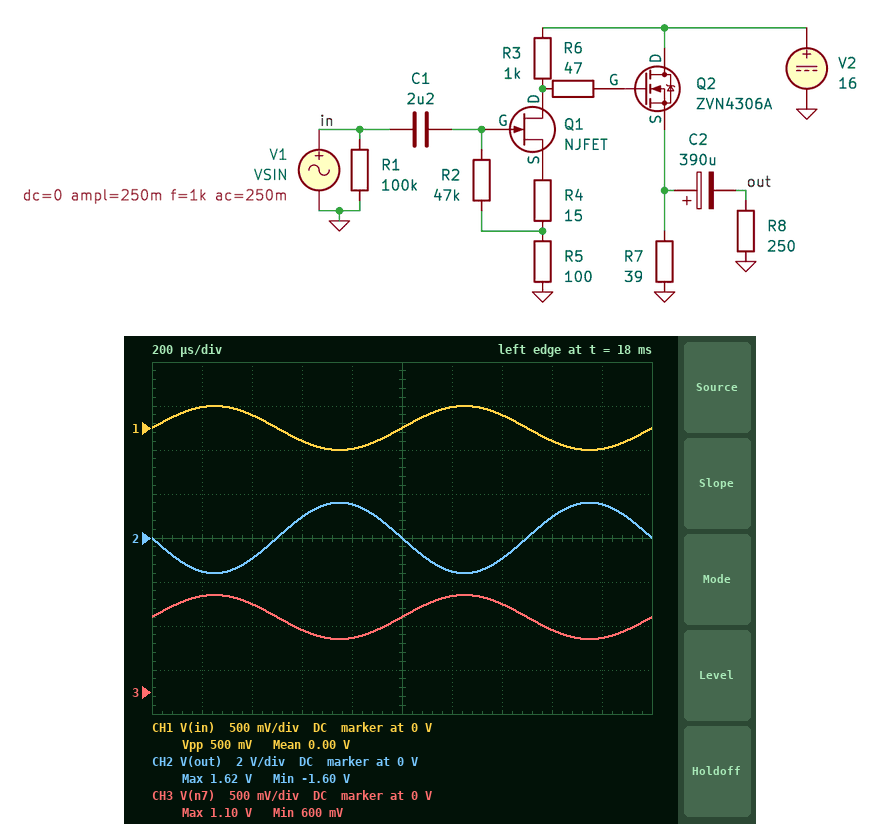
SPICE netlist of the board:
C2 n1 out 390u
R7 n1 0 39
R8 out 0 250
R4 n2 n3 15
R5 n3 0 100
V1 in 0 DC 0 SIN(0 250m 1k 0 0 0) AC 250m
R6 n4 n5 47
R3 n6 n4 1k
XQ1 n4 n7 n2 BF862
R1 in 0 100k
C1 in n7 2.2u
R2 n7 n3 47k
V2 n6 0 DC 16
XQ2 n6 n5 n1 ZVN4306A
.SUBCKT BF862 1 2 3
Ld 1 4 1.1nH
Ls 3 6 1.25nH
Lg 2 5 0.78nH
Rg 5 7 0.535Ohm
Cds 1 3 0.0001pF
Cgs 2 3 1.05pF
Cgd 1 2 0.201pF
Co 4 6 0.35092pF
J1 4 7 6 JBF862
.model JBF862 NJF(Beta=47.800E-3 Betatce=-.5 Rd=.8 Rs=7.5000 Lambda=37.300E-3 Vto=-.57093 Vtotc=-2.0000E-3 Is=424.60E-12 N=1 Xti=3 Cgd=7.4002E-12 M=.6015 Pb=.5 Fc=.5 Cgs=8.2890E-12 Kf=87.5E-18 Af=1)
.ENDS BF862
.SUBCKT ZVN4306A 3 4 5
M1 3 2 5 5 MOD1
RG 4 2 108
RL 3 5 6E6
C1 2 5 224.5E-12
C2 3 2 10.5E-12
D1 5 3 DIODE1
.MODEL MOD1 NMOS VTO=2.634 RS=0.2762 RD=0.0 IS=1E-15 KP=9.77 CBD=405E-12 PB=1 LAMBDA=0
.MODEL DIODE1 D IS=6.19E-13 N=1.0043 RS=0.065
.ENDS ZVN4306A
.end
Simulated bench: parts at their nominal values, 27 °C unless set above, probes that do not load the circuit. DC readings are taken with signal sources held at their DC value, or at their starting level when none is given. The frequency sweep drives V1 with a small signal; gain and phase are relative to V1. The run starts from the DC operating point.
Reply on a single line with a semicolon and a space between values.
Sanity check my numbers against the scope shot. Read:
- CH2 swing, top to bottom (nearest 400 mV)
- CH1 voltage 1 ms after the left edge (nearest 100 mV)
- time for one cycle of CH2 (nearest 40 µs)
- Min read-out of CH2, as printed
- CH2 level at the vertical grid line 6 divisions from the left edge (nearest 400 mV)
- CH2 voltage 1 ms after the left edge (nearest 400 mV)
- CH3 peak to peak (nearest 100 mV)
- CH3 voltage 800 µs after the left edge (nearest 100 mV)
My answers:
3.2 V; 0 V; 1.00 ms; -1.60 V; -1.6 V; 0 V; 500 mV; 600 mV
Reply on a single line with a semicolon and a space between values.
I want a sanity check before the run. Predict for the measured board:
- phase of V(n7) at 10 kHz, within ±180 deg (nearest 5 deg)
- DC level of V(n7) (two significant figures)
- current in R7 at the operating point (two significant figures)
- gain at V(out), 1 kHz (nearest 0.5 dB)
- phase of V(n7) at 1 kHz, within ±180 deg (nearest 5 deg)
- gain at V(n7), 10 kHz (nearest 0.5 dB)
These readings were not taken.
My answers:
0 deg; 850 mV; 120 mA; 16.0 dB; 0 deg; 0 dB
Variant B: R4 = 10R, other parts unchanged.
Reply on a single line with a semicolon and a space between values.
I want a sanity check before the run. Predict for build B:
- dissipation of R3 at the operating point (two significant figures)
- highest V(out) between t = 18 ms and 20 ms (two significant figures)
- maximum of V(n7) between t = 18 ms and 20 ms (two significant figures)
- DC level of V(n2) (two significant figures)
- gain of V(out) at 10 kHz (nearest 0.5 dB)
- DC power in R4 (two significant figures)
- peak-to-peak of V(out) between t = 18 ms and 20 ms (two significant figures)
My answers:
89 mW; 1.7 V; 1.2 V; 1.0 V; 16.5 dB; 890 µW; 3.3 V
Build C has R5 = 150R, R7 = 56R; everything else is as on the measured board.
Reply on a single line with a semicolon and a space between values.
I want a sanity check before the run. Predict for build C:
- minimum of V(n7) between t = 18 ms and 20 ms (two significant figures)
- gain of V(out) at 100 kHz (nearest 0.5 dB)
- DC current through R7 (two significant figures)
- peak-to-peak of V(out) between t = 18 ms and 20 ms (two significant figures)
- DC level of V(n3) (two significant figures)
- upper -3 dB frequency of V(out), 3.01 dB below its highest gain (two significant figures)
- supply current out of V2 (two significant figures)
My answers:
1.0 V; 13.5 dB; 85 mA; 2.4 V; 1.3 V; 8.8 MHz; 93 mA
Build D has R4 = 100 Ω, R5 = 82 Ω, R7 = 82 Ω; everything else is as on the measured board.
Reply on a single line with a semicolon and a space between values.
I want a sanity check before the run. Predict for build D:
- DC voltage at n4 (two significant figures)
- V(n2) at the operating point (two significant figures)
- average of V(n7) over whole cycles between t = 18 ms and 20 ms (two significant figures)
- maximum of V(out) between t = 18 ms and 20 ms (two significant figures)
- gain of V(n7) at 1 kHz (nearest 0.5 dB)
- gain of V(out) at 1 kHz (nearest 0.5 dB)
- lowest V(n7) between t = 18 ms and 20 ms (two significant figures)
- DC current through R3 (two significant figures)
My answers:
13 V; 600 mV; 270 mV; 1.1 V; 0 dB; 13.0 dB; 19 mV; 3.3 mA
